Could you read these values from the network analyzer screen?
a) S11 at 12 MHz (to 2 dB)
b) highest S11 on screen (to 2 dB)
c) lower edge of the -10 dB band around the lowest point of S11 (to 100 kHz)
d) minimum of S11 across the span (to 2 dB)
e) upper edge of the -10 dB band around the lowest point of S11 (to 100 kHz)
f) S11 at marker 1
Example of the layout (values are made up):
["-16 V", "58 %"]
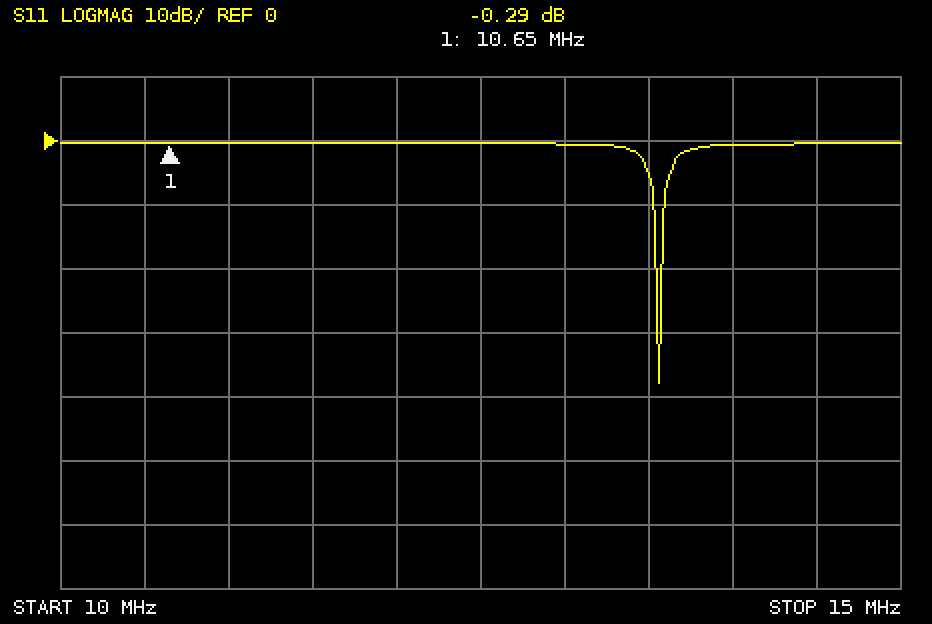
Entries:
["0 dB", "0 dB", "13.5 MHz", "-38 dB", "13.6 MHz", "-0.29 dB"]
